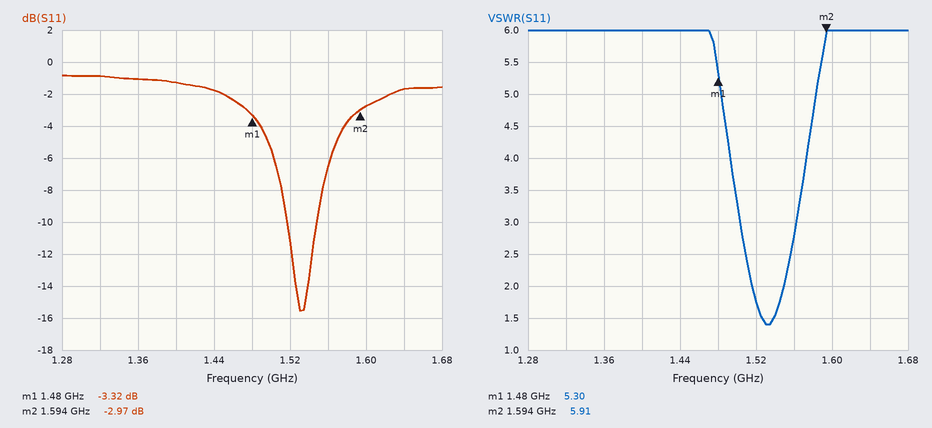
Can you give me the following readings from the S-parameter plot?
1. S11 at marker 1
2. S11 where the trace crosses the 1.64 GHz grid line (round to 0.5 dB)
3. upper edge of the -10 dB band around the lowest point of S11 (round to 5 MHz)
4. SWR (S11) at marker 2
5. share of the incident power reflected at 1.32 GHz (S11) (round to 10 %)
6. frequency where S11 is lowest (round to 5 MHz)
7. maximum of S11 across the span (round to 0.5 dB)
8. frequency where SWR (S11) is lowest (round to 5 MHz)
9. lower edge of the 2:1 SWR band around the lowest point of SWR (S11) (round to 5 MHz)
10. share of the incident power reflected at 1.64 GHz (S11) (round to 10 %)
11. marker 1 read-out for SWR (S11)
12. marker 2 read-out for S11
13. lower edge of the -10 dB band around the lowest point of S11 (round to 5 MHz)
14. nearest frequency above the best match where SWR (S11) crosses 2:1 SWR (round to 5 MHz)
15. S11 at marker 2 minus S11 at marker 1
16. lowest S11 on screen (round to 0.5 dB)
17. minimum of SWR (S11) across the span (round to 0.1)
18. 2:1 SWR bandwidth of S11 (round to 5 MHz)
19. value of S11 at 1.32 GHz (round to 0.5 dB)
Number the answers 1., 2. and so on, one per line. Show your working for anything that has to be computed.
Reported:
1. -3.32 dB
2. -1.5 dB
3. 1.550 GHz
4. 5.91
5. 10^(-1/10) ≈ 79.4 %, so 80 % to the nearest 10 %
6. 1.530 GHz
7. -1.0 dB
8. 1.530 GHz
9. 1.515 GHz
10. 10^(-1.5/10) ≈ 70.8 %, so 70 % to the nearest 10 %
11. 5.30
12. -2.97 dB
13. 1.515 GHz
14. 1.550 GHz
15. -2.97 − (-3.32) = 0.35 dB
16. -15.5 dB
17. 1.4
18. 1.550 GHz − 1.515 GHz = 35 MHz
19. -1.0 dB
